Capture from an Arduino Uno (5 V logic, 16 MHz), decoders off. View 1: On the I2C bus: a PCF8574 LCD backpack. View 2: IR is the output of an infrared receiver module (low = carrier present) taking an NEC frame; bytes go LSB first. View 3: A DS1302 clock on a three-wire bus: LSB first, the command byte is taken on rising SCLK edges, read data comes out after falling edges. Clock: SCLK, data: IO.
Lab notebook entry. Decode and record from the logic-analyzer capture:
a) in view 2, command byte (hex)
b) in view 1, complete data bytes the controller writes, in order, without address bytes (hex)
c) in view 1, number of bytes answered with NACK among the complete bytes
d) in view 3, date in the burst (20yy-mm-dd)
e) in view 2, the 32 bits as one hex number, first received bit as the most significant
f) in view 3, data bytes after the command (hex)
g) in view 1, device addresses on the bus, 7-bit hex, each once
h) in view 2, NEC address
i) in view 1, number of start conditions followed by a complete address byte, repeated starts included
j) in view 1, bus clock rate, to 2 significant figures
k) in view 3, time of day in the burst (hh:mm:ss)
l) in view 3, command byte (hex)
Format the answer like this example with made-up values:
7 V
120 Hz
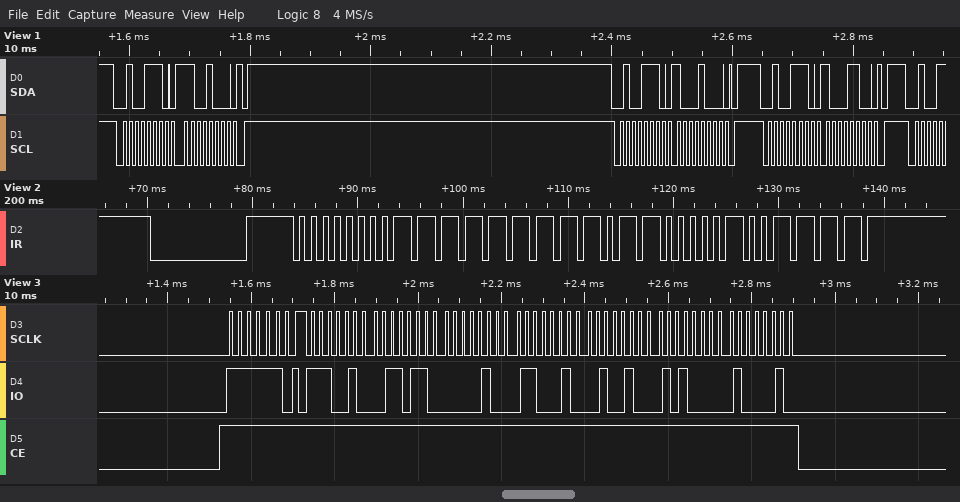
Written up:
0x0D
C8 88 8C
0
2021-12-23
0x00FFB04F
27 36 10 23 12 05 21
0x27
0x00
3
100 kHz
10:36:27
0xBF
